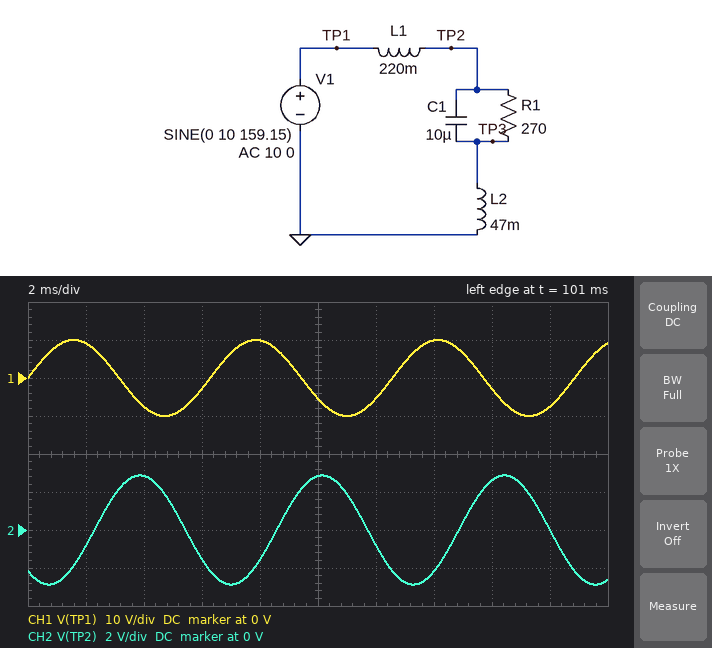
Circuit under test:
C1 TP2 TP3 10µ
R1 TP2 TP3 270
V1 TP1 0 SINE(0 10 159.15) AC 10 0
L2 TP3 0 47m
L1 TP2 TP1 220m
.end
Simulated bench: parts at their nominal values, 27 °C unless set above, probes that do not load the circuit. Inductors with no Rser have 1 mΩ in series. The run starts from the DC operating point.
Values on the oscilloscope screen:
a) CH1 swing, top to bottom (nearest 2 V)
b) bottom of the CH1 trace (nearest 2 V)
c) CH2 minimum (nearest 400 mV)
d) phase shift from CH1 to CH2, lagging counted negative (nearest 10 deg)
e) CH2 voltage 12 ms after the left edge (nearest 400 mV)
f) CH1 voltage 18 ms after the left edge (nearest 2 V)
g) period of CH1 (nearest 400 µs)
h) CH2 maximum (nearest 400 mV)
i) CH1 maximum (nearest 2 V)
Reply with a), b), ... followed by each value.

a) 20 V
b) -10 V
c) -2.8 V
d) -130 deg
e) -800 mV
f) -8 V
g) 6.4 ms
h) 2.8 V
i) 10 V
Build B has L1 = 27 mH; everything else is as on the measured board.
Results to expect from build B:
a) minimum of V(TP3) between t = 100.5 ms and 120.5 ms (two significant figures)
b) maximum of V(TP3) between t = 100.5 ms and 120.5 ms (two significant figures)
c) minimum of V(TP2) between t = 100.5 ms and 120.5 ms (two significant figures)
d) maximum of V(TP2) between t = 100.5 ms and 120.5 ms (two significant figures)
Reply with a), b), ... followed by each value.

a) -13 V
b) 13 V
c) -15 V
d) 15 V
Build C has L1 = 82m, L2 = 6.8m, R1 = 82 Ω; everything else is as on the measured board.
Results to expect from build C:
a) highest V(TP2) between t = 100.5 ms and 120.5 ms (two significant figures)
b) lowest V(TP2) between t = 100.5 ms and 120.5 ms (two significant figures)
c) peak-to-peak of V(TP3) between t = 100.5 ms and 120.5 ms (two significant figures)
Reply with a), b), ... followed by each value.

a) 8.6 V
b) -8.6 V
c) 2.0 V
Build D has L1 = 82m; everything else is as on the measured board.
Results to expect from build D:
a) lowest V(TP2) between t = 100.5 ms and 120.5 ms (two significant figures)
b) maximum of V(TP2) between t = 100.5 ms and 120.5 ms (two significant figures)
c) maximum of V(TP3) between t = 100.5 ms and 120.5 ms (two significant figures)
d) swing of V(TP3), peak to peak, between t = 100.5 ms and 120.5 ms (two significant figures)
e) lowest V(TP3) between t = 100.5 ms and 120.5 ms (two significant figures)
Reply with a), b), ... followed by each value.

a) -10 V
b) 10 V
c) 9.0 V
d) 18 V
e) -9.0 V
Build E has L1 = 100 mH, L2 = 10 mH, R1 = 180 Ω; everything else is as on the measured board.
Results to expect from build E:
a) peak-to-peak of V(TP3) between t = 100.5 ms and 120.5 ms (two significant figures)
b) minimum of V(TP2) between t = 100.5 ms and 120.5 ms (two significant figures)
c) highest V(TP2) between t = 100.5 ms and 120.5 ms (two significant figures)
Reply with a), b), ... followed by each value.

a) 3.7 V
b) -15 V
c) 15 V
